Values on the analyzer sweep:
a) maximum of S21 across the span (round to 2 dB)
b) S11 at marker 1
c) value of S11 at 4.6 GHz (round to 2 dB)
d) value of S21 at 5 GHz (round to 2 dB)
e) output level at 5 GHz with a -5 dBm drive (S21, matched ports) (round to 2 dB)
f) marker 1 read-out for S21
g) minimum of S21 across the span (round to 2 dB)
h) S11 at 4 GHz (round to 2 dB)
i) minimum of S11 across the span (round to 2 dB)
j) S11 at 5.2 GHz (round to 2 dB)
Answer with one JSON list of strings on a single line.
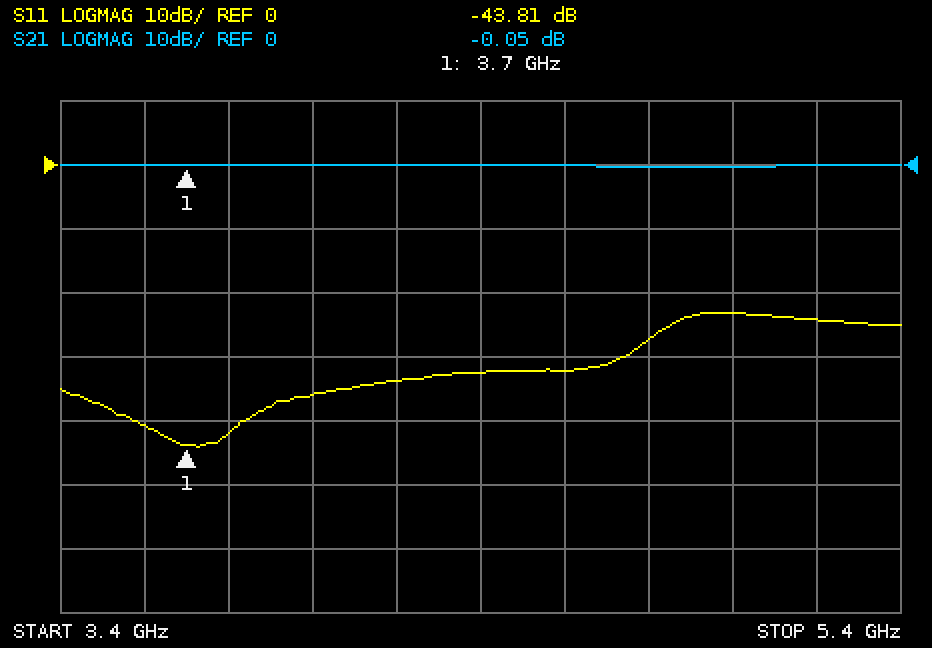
["0 dB", "-43.81 dB", "-32 dB", "0 dB", "-6 dBm", "-0.05 dB", "0 dB", "-36 dB", "-44 dB", "-24 dB"]
